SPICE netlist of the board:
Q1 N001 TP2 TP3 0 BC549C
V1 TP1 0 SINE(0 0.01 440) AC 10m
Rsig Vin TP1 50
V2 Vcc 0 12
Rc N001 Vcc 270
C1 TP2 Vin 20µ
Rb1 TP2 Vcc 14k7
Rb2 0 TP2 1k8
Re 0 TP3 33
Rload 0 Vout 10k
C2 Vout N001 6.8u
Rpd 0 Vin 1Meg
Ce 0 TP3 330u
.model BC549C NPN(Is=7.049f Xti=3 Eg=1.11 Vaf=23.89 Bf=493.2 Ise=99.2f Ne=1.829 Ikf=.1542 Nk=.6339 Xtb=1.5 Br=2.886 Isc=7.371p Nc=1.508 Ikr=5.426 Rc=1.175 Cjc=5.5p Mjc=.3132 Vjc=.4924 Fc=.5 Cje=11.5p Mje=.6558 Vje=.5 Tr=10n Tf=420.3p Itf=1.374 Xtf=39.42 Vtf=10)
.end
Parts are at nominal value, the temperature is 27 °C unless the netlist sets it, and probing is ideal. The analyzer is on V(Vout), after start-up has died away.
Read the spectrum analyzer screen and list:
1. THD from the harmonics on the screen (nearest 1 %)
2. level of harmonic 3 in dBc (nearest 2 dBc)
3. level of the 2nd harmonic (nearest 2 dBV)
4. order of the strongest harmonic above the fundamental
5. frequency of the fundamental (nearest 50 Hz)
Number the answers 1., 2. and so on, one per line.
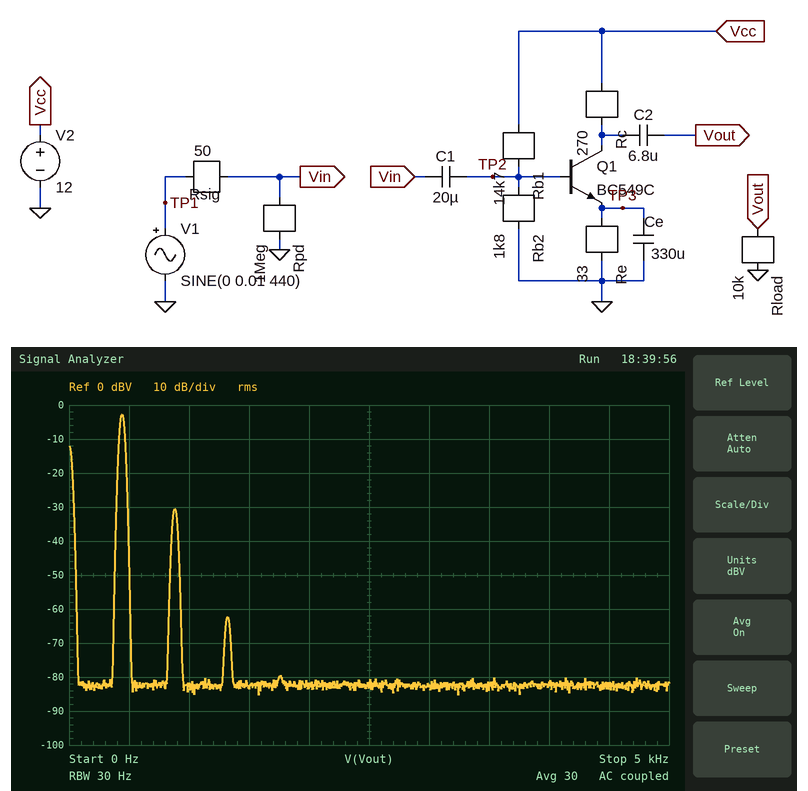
1. 4 %
2. -60 dBc
3. -30 dBV
4. 2
5. 450 Hz
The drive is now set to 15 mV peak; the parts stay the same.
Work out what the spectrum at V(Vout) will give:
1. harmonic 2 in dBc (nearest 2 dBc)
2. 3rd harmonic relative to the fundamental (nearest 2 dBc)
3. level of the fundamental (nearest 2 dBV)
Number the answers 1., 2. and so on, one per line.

1. -24 dBc
2. -52 dBc
3. 0 dBV
